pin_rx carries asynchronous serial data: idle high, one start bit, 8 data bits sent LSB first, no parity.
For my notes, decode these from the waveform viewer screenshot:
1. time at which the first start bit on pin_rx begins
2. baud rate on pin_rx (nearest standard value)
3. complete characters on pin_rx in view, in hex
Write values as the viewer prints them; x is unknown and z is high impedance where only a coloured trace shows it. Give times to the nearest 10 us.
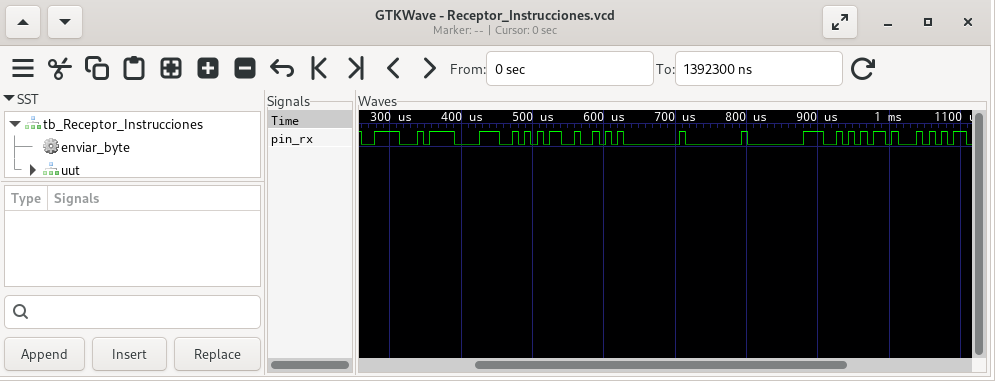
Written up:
260 us
115200 baud
1E, 0F, AA, 52, 00, 00, 00, AA, 51
